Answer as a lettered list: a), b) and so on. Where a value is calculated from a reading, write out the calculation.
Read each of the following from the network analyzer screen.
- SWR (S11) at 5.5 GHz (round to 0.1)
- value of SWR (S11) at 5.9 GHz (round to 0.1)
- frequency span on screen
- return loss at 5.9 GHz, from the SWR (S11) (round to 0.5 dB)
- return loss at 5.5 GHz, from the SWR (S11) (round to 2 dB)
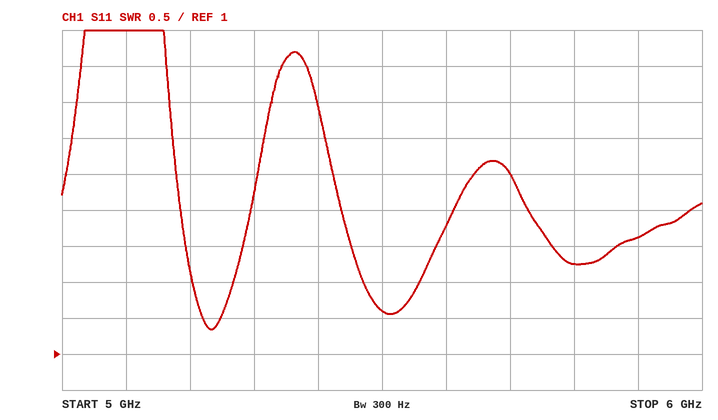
a) 1.6
b) 2.6
c) 1 GHz
d) −20 log10((2.6 − 1)/(2.6 + 1)) ≈ 7.0 dB
e) −20 log10((1.6 − 1)/(1.6 + 1)) ≈ 12.7 dB, so 12 dB to the nearest 2 dB
